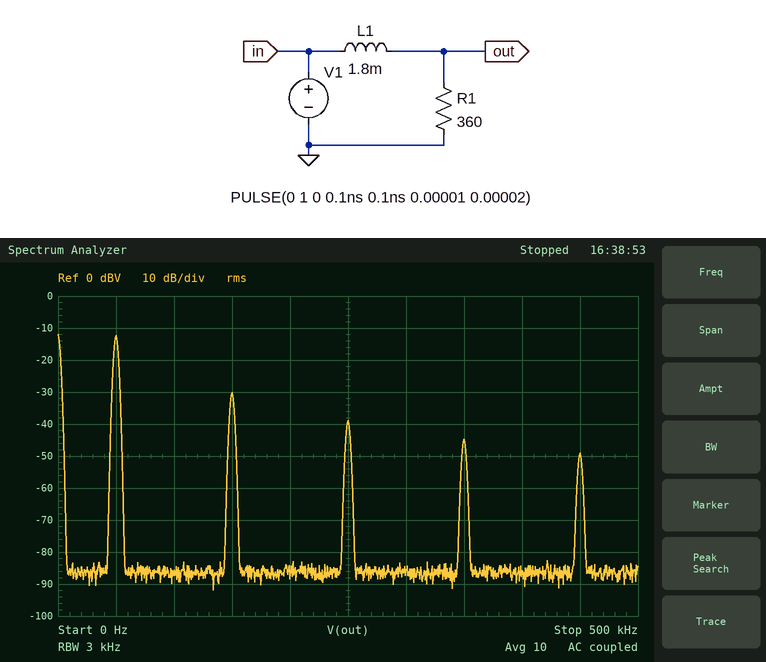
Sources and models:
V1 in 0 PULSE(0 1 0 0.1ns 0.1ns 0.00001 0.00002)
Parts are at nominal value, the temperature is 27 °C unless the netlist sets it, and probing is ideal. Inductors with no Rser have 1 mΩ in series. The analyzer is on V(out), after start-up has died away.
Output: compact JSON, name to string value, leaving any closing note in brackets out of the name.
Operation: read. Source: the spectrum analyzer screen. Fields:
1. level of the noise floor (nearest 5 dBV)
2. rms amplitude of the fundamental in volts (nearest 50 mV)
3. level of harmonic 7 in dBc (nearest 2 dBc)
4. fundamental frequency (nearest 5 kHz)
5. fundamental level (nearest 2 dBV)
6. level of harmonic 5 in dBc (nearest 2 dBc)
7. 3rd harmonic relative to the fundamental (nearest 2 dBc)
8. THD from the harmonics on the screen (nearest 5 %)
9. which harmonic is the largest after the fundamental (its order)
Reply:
{"level of the noise floor": "-85 dBV", "rms amplitude of the fundamental in volts": "250 mV", "level of harmonic 7 in dBc": "-32 dBc", "fundamental frequency": "50 kHz", "fundamental level": "-12 dBV", "level of harmonic 5 in dBc": "-26 dBc", "3rd harmonic relative to the fundamental": "-18 dBc", "THD from the harmonics on the screen": "15 %", "which harmonic is the largest after the fundamental": "3"}
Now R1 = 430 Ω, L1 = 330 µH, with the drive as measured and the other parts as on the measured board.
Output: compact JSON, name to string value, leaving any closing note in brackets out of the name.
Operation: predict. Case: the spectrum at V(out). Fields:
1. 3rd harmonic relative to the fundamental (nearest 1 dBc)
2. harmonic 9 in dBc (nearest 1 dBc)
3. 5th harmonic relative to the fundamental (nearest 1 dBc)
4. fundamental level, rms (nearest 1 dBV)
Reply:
{"3rd harmonic relative to the fundamental": "-11 dBc", "harmonic 9 in dBc": "-26 dBc", "5th harmonic relative to the fundamental": "-18 dBc", "fundamental level, rms": "-7 dBV"}
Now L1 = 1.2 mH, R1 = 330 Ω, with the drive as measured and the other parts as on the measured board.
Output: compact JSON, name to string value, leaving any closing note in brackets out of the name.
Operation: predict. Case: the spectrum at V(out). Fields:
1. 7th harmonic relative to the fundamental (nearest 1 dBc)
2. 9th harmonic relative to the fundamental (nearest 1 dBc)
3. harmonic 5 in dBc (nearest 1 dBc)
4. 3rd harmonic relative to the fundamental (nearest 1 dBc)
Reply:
{"7th harmonic relative to the fundamental": "-31 dBc", "9th harmonic relative to the fundamental": "-36 dBc", "harmonic 5 in dBc": "-26 dBc", "3rd harmonic relative to the fundamental": "-17 dBc"}
